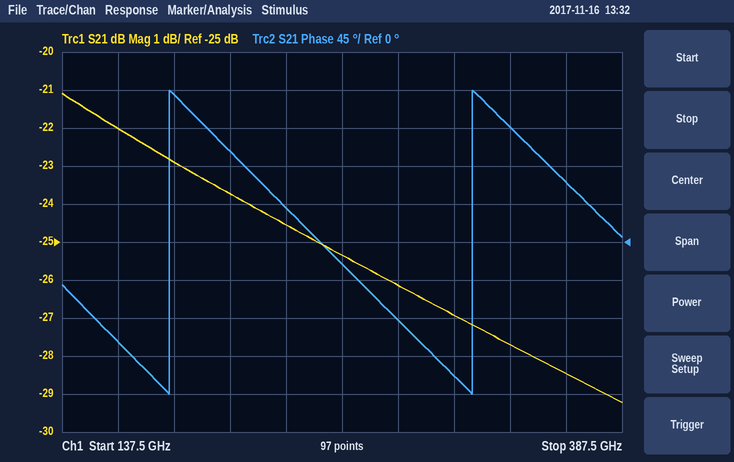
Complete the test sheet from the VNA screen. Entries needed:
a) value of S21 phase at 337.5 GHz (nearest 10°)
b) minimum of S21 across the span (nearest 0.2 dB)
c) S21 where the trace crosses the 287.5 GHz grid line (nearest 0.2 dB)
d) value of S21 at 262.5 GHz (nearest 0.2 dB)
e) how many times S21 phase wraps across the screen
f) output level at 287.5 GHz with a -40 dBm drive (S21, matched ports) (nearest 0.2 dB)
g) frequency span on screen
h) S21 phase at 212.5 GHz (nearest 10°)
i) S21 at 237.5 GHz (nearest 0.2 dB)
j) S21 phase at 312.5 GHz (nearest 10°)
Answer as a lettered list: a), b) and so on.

a) 140°
b) -29.2 dB
c) -26.2 dB
d) -25.4 dB
e) 2
f) -66.2 dBm
g) 250 GHz
h) 110°
i) -24.6 dB
j) -160°
